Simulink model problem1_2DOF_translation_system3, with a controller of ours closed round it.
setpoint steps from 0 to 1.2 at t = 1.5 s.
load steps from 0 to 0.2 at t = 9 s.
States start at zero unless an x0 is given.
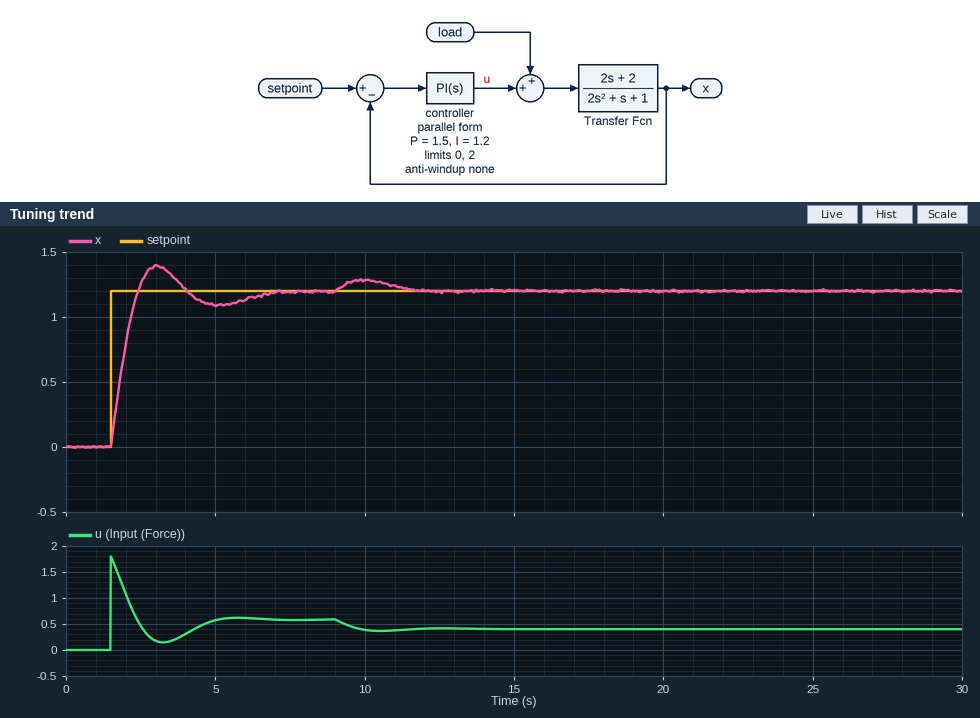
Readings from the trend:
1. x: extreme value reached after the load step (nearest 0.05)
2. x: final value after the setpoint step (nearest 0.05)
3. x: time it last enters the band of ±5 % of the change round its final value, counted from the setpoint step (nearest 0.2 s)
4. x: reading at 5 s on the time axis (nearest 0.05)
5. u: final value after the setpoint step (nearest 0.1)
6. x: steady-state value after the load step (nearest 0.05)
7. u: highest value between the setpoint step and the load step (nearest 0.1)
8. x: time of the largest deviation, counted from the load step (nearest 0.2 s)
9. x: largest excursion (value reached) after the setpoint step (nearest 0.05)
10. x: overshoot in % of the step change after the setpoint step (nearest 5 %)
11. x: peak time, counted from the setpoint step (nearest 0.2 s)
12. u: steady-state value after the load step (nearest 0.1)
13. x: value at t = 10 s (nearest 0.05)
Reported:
1.30
1.20
4.6 s
1.10
0.6
1.20
1.8
1.0 s
1.40
15 %
1.6 s
0.4
1.30
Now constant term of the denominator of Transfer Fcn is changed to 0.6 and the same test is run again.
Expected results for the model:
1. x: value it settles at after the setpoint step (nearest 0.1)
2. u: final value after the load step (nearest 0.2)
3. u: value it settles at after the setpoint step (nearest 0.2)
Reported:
1.2
0.2
0.4
